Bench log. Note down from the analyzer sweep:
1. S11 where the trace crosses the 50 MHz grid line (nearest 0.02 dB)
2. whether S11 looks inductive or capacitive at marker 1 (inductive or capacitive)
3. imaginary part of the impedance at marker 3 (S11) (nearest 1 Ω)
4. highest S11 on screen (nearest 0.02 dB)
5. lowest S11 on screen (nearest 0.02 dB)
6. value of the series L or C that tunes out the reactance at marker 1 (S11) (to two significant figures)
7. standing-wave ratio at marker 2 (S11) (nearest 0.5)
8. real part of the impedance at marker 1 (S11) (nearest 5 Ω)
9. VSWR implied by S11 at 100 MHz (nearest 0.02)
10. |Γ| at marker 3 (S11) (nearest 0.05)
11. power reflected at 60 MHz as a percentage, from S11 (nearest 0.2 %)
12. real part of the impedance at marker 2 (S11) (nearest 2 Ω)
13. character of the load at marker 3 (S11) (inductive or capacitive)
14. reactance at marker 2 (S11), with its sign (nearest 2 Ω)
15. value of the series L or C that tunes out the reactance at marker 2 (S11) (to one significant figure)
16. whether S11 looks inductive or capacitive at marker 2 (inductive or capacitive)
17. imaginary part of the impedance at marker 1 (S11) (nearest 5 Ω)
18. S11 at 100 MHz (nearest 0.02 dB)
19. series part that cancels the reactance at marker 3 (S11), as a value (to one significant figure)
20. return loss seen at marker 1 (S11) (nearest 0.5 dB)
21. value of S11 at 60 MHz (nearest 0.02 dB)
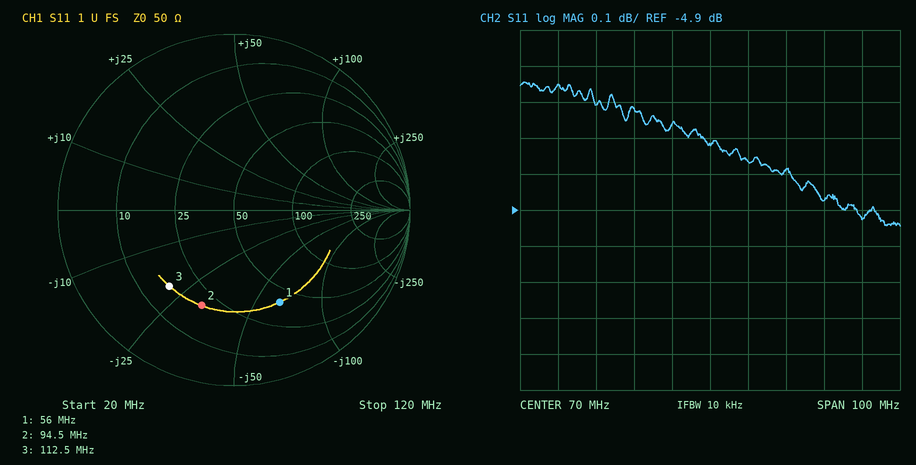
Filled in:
-4.62 dB
capacitive
-21 Ω
-4.54 dB
-4.94 dB
180 nH
3.5
40 Ω
3.66
0.55
34.2 %
20 Ω
capacitive
-32 Ω
50 nH
capacitive
-65 Ω
-4.88 dB
30 nH
4.5 dB
-4.66 dB
